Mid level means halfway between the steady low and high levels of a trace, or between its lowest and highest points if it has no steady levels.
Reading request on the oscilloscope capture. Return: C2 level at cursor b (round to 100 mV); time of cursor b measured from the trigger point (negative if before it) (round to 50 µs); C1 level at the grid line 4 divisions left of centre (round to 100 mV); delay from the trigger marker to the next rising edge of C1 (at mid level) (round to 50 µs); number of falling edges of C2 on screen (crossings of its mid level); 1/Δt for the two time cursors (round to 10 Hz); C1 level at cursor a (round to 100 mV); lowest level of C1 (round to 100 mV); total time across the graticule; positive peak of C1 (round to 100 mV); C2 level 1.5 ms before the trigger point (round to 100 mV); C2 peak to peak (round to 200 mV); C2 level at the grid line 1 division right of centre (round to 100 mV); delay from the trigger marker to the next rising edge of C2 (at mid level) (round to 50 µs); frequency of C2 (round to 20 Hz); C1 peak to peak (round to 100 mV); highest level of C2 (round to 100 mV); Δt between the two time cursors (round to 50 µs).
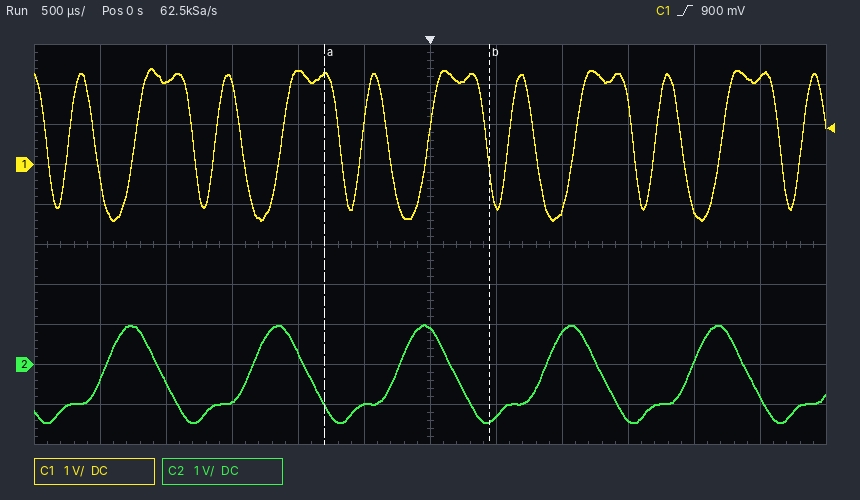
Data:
-1.4 V
+450 µs
2.1 V
600 µs
5
800 Hz
2.3 V
-1.4 V
6 ms
2.4 V
-900 mV
2.4 V
-1.3 V
850 µs
900 Hz
3.8 V
1.0 V
1.25 ms
